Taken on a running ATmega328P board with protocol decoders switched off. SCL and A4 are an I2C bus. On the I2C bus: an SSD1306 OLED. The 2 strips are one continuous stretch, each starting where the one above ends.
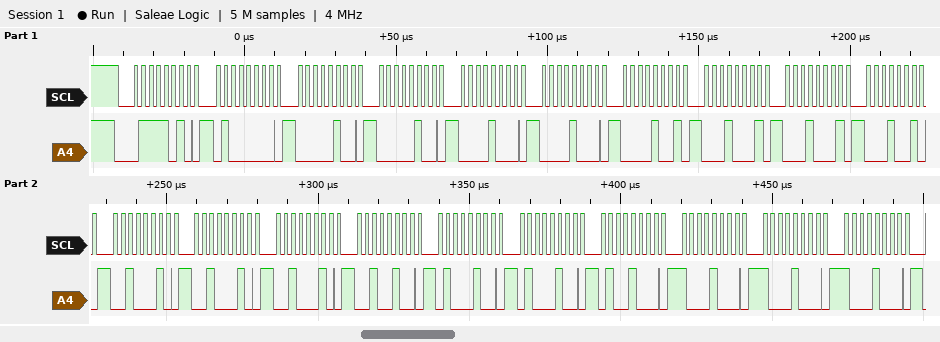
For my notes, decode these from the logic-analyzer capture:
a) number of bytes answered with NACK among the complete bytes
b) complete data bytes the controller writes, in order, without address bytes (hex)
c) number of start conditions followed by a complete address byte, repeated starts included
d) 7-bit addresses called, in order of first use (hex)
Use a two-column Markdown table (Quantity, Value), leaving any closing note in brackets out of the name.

| Quantity | Value |
|---|---|
| number of bytes answered with NACK among the complete bytes | 0 |
| complete data bytes the controller writes, in order, without address bytes | 40 04 04 08 08 09 11 11 12 22 22 22 24 44 44 48 88 88 88 |
| number of start conditions followed by a complete address byte, repeated starts included | 1 |
| 7-bit addresses called, in order of first use | 0x3D |
